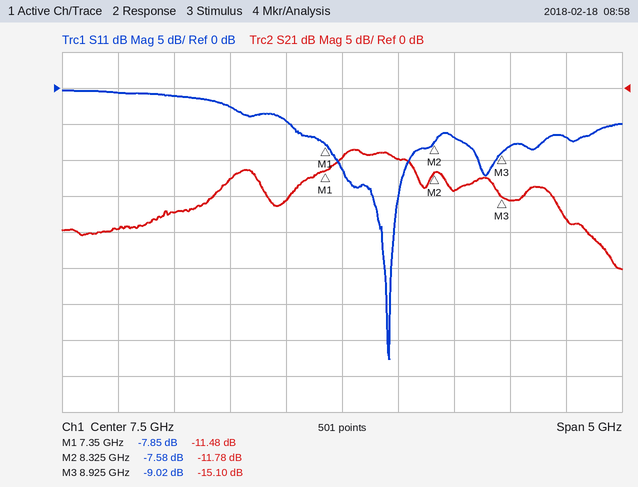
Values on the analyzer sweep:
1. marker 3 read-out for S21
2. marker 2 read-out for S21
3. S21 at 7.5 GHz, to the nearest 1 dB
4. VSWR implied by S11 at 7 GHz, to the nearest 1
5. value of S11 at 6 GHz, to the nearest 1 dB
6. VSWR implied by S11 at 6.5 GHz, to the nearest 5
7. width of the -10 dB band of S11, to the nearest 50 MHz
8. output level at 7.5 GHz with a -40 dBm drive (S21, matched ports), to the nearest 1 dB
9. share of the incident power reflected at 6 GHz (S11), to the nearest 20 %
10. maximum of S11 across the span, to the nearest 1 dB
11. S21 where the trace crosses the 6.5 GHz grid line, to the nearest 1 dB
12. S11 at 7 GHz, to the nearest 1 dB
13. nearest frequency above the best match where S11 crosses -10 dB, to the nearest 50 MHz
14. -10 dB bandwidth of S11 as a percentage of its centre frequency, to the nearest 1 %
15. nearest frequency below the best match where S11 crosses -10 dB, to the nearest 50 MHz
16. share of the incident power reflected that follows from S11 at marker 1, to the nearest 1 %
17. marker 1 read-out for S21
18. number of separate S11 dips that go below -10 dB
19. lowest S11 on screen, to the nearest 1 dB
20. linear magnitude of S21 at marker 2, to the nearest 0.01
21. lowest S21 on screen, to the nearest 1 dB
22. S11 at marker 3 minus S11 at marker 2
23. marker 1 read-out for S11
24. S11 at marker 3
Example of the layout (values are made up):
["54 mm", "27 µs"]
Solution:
["-15.10 dB", "-11.78 dB", "-10 dB", "4", "-1 dB", "5", "650 MHz", "-50 dBm", "80 %", "0 dB", "-13 dB", "-5 dB", "8.10 GHz", "8 %", "7.45 GHz", "16 %", "-11.48 dB", "2", "-38 dB", "0.26", "-25 dB", "-1.44 dB", "-7.85 dB", "-9.02 dB"]
